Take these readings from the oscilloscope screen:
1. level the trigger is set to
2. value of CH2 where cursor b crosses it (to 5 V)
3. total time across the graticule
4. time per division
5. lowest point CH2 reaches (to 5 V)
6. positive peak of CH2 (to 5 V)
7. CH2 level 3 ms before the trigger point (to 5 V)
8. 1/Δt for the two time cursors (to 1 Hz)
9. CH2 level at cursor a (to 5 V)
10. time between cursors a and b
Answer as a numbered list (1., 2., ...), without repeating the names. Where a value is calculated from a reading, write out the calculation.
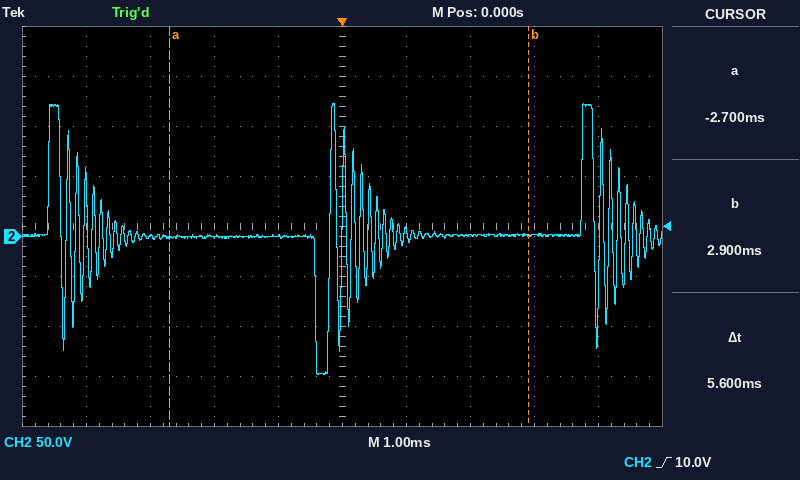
1. 10.0 V
2. 0 V
3. 10 ms
4. 1 ms
5. -140 V
6. 135 V
7. 0 V
8. 1 / 5.6 ms ≈ 179 Hz
9. 0 V
10. 5.6 ms
